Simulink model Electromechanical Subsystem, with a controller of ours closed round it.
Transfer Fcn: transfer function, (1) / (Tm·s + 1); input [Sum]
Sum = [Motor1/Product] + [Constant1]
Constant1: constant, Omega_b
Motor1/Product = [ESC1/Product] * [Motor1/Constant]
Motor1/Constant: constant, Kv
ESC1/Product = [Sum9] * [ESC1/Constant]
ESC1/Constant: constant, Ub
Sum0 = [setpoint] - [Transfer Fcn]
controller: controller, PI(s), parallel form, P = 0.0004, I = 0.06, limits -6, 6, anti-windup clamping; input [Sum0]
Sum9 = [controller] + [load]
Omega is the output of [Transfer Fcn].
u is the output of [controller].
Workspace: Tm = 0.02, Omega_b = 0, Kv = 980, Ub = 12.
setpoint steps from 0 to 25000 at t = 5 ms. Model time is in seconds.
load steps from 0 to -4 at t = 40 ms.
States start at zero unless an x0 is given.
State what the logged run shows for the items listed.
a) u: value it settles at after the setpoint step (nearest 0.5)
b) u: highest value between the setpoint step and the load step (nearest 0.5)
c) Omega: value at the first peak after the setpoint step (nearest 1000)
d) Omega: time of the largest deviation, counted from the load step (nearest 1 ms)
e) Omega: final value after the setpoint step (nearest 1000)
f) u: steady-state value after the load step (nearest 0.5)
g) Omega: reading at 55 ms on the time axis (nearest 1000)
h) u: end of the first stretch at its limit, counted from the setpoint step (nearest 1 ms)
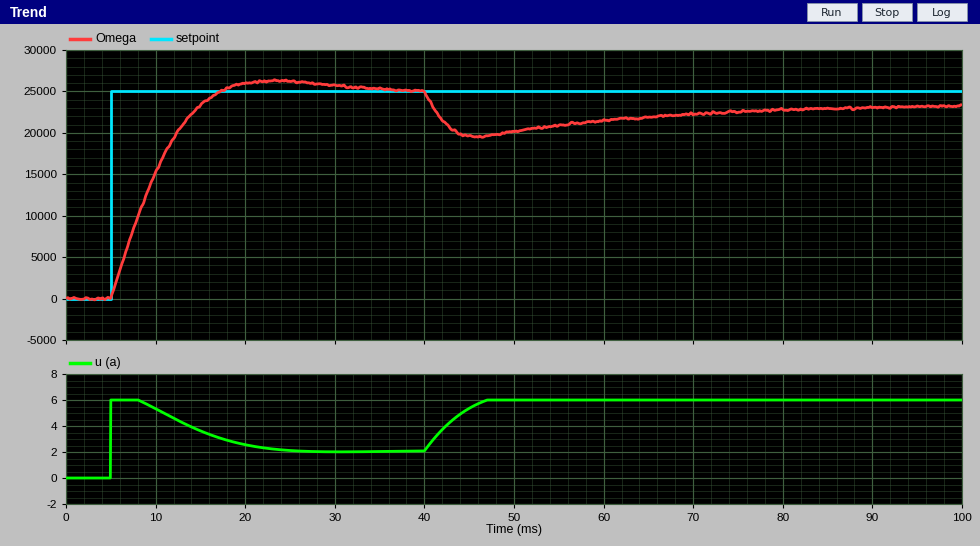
2.0
6.0
26000
6 ms
25000
6.0
21000
3 ms
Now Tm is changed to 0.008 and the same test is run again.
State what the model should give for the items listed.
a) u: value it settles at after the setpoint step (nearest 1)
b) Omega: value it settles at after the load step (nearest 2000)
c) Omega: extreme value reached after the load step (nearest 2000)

2
24000
18000
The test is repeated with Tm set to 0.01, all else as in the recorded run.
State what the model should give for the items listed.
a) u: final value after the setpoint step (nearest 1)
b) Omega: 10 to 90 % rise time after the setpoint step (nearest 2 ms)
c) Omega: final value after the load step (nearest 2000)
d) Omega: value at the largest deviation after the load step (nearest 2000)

2
6 ms
24000
18000
